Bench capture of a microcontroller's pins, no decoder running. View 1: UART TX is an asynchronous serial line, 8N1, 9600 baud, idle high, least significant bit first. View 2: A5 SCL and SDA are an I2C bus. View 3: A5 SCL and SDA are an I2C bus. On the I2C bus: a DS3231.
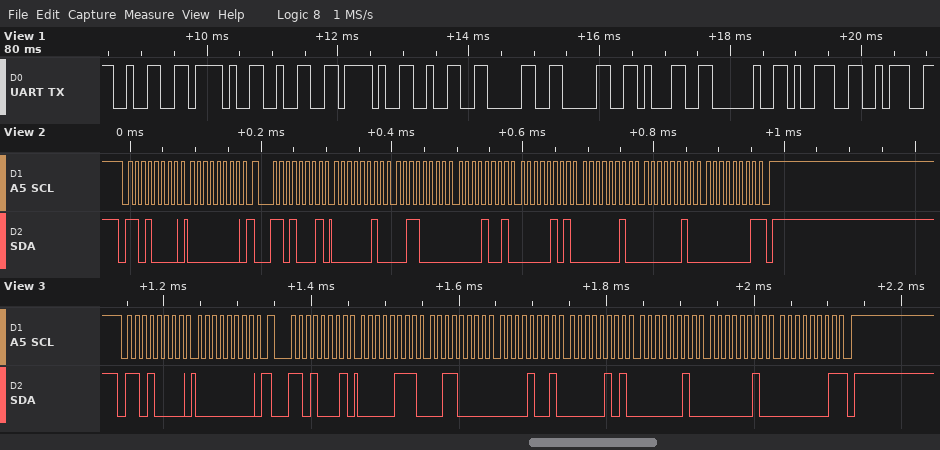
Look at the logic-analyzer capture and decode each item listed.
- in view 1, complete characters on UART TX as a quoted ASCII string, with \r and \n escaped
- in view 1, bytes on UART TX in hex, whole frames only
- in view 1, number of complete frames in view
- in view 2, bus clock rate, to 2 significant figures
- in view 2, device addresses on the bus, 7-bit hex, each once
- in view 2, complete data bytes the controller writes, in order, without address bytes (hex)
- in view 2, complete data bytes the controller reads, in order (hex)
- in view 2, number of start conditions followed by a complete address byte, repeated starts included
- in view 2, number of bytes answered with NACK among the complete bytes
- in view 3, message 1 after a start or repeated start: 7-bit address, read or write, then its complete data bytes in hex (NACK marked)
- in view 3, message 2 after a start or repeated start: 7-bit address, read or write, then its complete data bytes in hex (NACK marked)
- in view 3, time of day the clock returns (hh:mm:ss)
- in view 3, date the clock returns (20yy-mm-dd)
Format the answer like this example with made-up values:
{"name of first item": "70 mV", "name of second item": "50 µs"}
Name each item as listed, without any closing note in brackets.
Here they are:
{"in view 1, complete characters on UART TX as a quoted ASCII string, with \\r and \\n escaped": "\"2/2/2001 9:\"", "in view 1, bytes on UART TX in hex, whole frames only": "32 2F 32 2F 32 30 30 31 20 39 3A", "in view 1, number of complete frames in view": "11", "in view 2, bus clock rate, to 2 significant figures": "100 kHz", "in view 2, device addresses on the bus, 7-bit hex, each once": "0x68", "in view 2, complete data bytes the controller writes, in order, without address bytes": "00", "in view 2, complete data bytes the controller reads, in order": "02 30 09 05 02 02 01", "in view 2, number of start conditions followed by a complete address byte, repeated starts included": "2", "in view 2, number of bytes answered with NACK among the complete bytes": "1", "in view 3, message 1 after a start or repeated start: 7-bit address, read or write, then its complete data bytes in hex": "0x68 write: 00", "in view 3, message 2 after a start or repeated start: 7-bit address, read or write, then its complete data bytes in hex": "0x68 read: 07 30 09 05 02 02 01 NACK", "in view 3, time of day the clock returns": "09:30:07", "in view 3, date the clock returns": "2001-02-02"}
